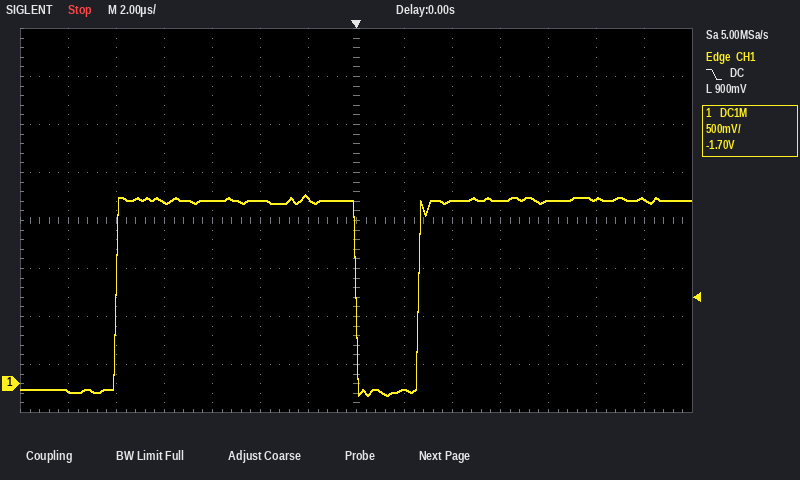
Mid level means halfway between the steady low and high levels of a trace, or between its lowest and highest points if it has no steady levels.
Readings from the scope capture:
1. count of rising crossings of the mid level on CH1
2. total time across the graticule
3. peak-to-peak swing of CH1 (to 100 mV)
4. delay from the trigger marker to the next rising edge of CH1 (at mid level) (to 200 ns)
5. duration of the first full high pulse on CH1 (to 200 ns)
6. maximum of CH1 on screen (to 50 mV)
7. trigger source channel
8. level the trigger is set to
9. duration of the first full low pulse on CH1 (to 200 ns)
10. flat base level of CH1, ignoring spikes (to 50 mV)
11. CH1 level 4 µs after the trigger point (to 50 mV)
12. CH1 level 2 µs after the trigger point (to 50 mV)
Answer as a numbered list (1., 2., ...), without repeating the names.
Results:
1. 2
2. 28 µs
3. 2.10 V
4. 2.6 µs
5. 10.0 µs
6. 1.95 V
7. CH1
8. 900 mV
9. 2.6 µs
10. -50 mV
11. 1.90 V
12. -50 mV
